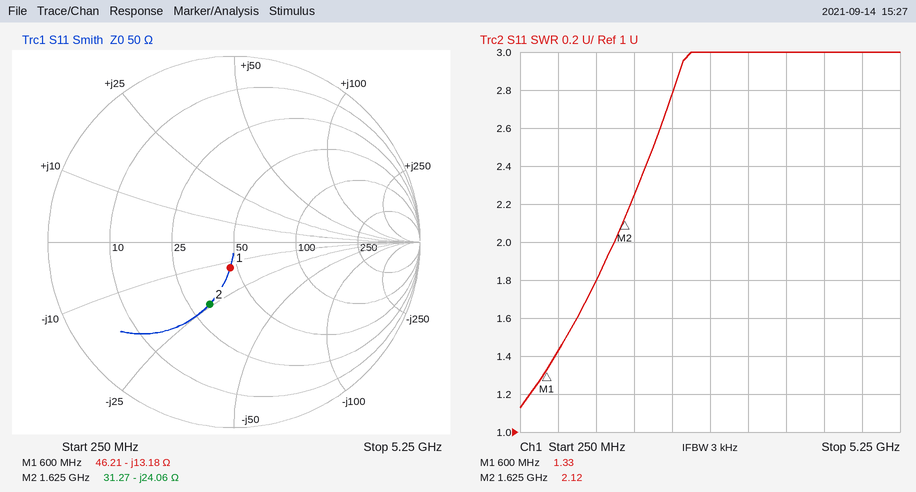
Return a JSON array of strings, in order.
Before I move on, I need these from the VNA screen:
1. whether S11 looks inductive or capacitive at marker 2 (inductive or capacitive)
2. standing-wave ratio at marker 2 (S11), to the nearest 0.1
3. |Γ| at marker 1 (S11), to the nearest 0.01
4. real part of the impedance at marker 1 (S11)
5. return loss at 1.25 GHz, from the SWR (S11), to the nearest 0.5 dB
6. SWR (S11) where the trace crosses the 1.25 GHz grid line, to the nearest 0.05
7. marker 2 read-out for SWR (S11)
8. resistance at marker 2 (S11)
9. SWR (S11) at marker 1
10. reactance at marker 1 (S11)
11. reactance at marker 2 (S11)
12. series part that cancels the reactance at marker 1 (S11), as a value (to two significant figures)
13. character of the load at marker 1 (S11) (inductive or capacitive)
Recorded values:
["capacitive", "2.1", "0.14", "46.21 Ω", "11.0 dB", "1.80", "2.12", "31.27 Ω", "1.33", "-13.18 Ω", "-24.06 Ω", "3.5 nH", "capacitive"]
